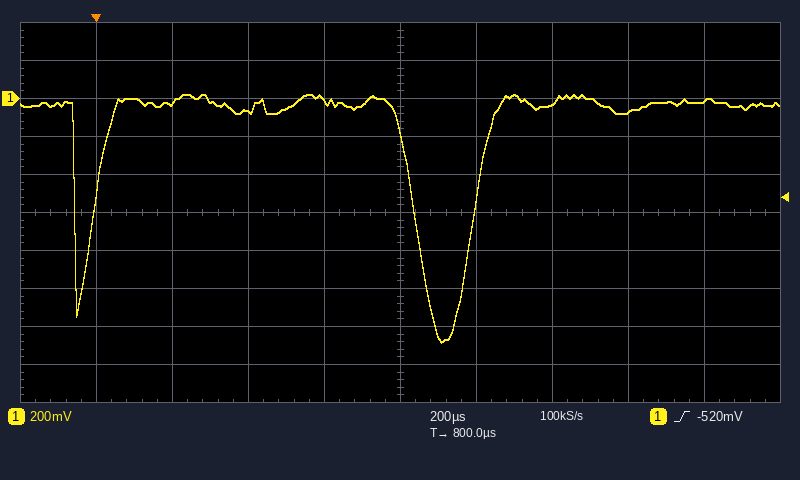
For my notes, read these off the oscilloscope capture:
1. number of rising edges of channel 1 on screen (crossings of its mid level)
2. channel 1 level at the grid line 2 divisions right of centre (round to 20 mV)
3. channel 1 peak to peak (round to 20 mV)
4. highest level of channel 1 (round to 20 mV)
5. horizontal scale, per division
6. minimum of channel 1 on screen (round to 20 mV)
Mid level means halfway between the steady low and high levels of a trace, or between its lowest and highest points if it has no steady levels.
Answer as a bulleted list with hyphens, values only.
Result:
- 2
- -20 mV
- 1.30 V
- 20 mV
- 200 µs
- -1.28 V
